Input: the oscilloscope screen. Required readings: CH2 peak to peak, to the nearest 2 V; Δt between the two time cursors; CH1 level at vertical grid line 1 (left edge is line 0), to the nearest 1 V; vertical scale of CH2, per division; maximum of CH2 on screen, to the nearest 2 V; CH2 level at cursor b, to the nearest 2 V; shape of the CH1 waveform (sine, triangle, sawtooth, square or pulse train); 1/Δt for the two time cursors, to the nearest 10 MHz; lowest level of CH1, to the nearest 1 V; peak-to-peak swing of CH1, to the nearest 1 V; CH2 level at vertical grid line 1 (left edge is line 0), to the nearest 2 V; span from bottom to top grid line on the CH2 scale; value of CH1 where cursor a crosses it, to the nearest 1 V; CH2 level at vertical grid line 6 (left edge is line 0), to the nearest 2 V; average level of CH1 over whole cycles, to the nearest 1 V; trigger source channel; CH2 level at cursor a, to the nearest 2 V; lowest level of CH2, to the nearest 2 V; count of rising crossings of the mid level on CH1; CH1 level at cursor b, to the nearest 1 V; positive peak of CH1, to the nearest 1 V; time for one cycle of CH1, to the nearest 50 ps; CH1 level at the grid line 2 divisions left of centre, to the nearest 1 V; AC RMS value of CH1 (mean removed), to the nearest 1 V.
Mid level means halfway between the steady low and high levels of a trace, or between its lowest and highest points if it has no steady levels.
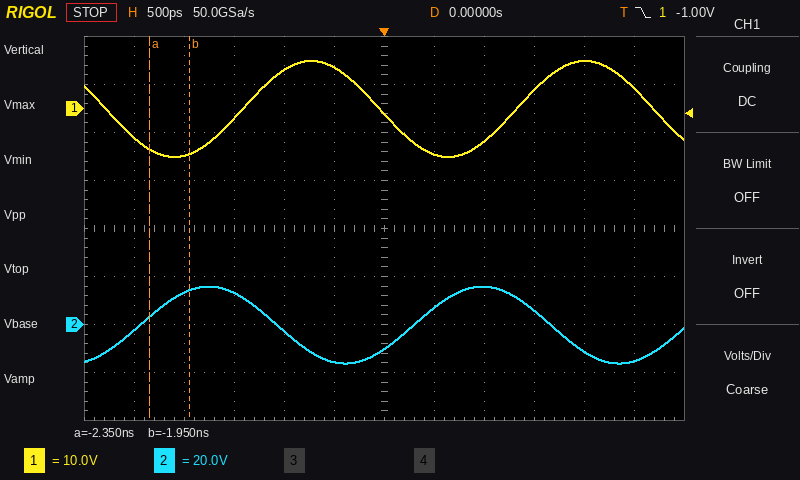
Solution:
32 V
400 ps
-6 V
20 V
16 V
14 V
sine
2.50 GHz
-10 V
20 V
-2 V
160 V
-8 V
-10 V
0 V
CH1
4 V
-16 V
2
-9 V
10 V
2.75 ns
8 V
7 V
